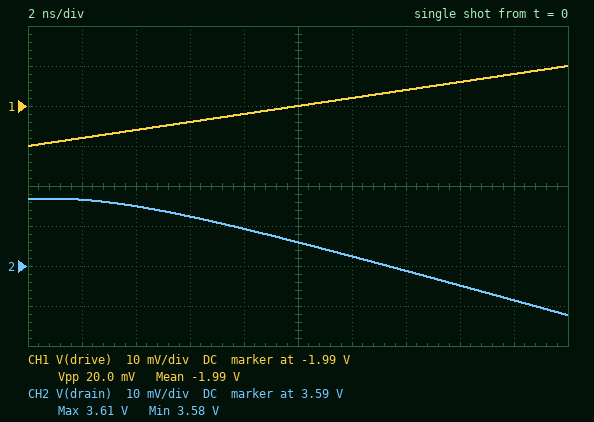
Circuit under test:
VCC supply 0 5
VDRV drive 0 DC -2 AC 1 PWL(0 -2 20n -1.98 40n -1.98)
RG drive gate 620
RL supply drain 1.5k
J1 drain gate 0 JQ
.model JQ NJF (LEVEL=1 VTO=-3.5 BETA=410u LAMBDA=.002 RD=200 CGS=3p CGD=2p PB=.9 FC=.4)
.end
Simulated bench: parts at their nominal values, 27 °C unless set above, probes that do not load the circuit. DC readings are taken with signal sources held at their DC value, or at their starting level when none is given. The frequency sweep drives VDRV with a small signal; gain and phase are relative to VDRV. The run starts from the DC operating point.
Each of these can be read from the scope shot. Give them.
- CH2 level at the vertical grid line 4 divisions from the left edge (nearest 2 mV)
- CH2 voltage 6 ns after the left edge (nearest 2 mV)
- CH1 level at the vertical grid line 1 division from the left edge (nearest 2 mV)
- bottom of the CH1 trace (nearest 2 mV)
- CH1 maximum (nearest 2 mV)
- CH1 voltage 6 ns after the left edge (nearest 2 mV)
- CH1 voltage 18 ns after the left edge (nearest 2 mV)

3.600 V
3.602 V
-1.998 V
-2.000 V
-1.980 V
-1.994 V
-1.982 V
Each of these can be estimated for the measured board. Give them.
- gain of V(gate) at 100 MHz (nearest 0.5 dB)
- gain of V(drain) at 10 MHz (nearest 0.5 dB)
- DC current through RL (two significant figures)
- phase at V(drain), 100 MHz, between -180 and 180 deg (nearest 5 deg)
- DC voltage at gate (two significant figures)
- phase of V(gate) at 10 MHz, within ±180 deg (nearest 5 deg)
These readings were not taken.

-5.5 dB
5.0 dB
930 µA
80 deg
-2.0 V
-10 deg
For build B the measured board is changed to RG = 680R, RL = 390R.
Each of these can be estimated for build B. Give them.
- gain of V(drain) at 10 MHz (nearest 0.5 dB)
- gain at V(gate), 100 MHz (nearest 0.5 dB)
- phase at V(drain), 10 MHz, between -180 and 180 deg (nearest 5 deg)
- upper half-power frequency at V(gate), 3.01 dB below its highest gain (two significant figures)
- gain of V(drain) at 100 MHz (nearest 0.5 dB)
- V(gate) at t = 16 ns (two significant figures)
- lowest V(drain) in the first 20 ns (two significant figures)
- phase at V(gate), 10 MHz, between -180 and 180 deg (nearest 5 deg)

-6.5 dB
-4.5 dB
170 deg
76 MHz
-10.5 dB
-2.0 V
4.6 V
-5 deg
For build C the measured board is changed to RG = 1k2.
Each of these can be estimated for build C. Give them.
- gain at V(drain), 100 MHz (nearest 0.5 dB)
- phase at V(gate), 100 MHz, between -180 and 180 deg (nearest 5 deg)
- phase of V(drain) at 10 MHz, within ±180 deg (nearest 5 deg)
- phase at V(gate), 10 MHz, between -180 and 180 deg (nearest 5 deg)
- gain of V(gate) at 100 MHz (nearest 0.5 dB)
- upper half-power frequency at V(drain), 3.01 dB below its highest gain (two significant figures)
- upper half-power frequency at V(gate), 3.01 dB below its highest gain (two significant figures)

-5.5 dB
-50 deg
155 deg
-15 deg
-9.5 dB
28 MHz
30 MHz
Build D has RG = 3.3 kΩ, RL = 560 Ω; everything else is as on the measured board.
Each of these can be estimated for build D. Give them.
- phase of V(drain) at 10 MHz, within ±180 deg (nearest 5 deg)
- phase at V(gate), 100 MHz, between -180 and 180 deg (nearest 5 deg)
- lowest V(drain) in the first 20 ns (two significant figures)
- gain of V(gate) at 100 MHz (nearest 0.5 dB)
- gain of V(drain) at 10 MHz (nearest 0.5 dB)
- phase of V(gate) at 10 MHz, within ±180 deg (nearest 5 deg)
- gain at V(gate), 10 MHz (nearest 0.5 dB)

145 deg
-75 deg
4.5 V
-16.0 dB
-4.5 dB
-30 deg
-1.5 dB
